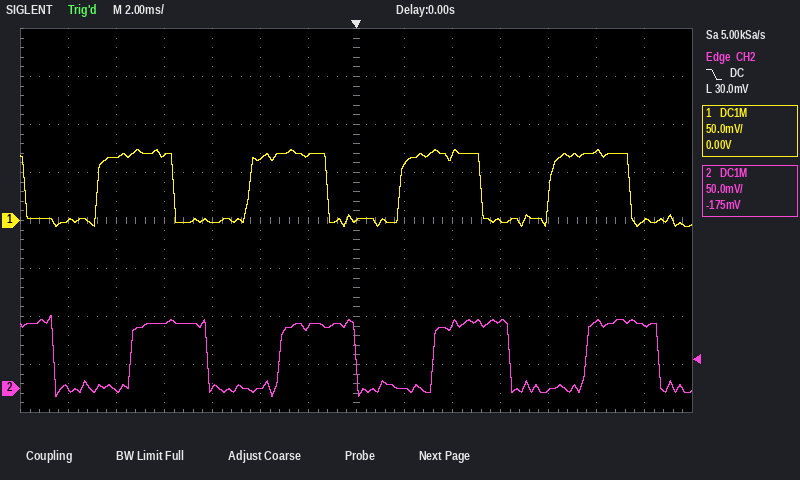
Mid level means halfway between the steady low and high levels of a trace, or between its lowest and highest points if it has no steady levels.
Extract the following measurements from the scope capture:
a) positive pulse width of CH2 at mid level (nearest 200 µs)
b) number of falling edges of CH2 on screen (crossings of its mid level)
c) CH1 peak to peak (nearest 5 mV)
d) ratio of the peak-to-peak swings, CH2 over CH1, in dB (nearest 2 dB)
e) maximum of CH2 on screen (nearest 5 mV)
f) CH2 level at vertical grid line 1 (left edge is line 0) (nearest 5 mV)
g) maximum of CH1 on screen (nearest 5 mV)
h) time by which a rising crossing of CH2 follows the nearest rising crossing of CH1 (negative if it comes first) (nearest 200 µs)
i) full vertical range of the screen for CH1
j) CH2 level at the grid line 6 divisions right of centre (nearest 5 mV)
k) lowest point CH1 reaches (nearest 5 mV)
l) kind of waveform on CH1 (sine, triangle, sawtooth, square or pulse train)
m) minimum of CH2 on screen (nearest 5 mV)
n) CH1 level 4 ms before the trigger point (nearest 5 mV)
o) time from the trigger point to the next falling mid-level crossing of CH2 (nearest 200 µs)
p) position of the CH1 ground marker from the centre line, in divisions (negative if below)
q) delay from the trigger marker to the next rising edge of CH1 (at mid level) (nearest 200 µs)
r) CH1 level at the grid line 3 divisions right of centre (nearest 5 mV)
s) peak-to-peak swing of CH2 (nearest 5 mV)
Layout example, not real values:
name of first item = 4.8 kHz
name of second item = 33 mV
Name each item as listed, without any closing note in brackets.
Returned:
positive pulse width of CH2 at mid level = 3.2 ms
number of falling edges of CH2 on screen = 5
CH1 peak to peak = 80 mV
ratio of the peak-to-peak swings, CH2 over CH1, in dB = 0 dB
maximum of CH2 on screen = 75 mV
CH2 level at vertical grid line 1 (left edge is line 0) = 0 mV
maximum of CH1 on screen = 75 mV
time by which a rising crossing of CH2 follows the nearest rising crossing of CH1 (negative if it comes first) = +1.4 ms
full vertical range of the screen for CH1 = 400 mV
CH2 level at the grid line 6 divisions right of centre = 65 mV
lowest point CH1 reaches = -5 mV
kind of waveform on CH1 = square
minimum of CH2 on screen = -10 mV
CH1 level 4 ms before the trigger point = 65 mV
time from the trigger point to the next falling mid-level crossing of CH2 = 6.4 ms
position of the CH1 ground marker from the centre line, in divisions = 0.0 div
delay from the trigger marker to the next rising edge of CH1 (at mid level) = 1.8 ms
CH1 level at the grid line 3 divisions right of centre = 0 mV
peak-to-peak swing of CH2 = 85 mV
